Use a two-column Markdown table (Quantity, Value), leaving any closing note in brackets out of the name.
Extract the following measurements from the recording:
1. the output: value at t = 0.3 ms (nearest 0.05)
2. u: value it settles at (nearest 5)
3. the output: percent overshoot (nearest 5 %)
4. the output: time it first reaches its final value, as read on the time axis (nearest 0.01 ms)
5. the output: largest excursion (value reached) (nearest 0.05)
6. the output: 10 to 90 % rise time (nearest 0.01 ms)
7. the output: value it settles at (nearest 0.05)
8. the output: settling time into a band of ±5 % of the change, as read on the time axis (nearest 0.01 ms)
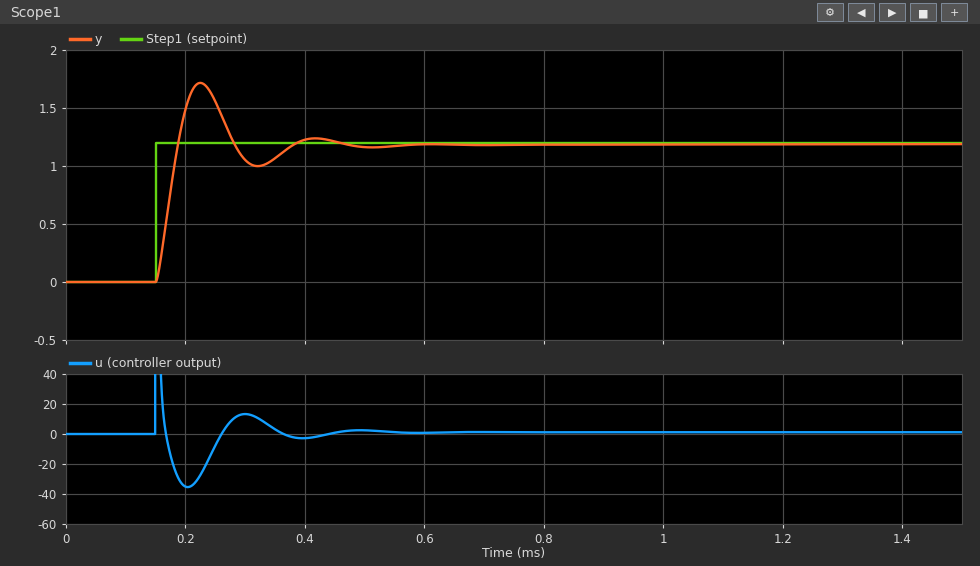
| Quantity | Value |
|---|---|
| the output: value at t = 0.3 ms | 1.05 |
| u: value it settles at | 0 |
| the output: percent overshoot | 45 % |
| the output: time it first reaches its final value, as read on the time axis | 0.19 ms |
| the output: largest excursion (value reached) | 1.70 |
| the output: 10 to 90 % rise time | 0.03 ms |
| the output: value it settles at | 1.20 |
| the output: settling time into a band of ±5 % of the change, as read on the time axis | 0.37 ms |
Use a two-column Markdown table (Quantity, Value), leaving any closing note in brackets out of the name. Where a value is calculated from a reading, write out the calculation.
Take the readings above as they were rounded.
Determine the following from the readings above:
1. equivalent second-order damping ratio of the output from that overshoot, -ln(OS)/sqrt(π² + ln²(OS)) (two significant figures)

| Quantity | Value |
|---|---|
| equivalent second-order damping ratio of the output from that overshoot, -ln(OS)/sqrt(π² + ln²(OS)) | ln(0.45) = -0.799; 0.799 / sqrt(9.870 + 0.638) = 0.25 |
